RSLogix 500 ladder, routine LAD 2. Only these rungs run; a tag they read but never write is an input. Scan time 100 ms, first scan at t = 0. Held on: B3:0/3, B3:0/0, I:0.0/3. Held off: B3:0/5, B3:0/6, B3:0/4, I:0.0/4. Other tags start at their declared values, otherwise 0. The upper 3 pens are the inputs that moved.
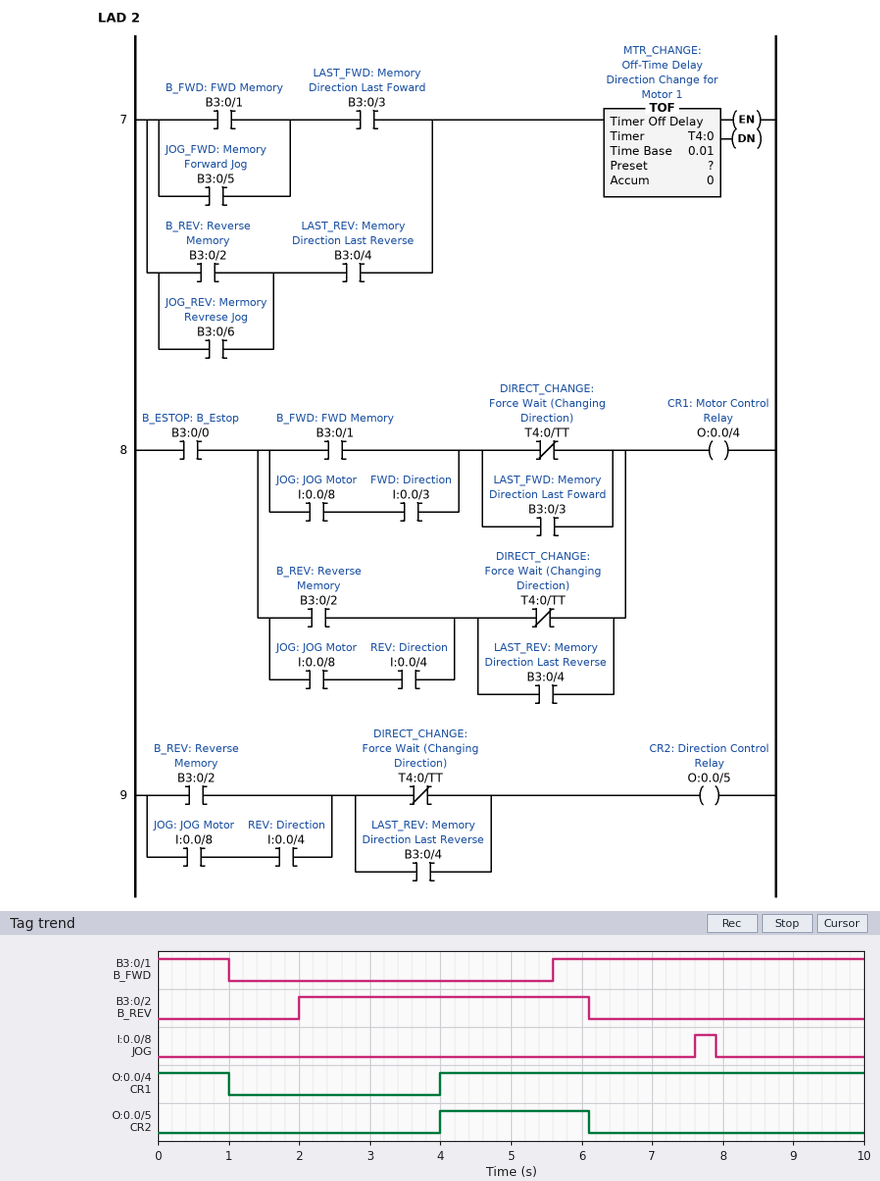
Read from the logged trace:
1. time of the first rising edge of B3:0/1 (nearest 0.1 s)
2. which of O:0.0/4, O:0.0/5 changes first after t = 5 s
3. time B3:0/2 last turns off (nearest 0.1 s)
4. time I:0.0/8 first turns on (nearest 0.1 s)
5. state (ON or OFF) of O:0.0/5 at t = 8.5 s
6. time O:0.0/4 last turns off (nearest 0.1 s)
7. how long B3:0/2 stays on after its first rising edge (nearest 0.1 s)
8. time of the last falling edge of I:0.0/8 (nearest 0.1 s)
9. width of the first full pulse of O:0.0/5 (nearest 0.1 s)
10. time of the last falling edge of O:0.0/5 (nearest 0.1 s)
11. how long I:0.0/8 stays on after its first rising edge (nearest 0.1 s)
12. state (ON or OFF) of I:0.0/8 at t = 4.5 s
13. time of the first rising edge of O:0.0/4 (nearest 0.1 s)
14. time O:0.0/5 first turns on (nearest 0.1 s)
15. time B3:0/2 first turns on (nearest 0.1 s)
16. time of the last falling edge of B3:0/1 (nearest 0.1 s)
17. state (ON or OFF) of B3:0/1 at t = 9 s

5.6 s
O:0.0/5
6.1 s
7.6 s
OFF
1.0 s
4.1 s
7.9 s
2.1 s
6.1 s
0.3 s
OFF
4.0 s
4.0 s
2.0 s
1.0 s
ON
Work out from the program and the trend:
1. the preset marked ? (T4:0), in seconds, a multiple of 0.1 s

3.0 s
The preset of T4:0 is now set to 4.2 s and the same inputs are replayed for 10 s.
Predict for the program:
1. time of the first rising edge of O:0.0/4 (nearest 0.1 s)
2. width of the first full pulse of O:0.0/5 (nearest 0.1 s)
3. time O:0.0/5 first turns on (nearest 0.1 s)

5.2 s
0.9 s
5.2 s
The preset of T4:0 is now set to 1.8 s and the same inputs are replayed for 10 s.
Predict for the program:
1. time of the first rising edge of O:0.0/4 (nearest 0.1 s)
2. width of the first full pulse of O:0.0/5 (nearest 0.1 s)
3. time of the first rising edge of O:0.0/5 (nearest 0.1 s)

2.8 s
3.3 s
2.8 s
